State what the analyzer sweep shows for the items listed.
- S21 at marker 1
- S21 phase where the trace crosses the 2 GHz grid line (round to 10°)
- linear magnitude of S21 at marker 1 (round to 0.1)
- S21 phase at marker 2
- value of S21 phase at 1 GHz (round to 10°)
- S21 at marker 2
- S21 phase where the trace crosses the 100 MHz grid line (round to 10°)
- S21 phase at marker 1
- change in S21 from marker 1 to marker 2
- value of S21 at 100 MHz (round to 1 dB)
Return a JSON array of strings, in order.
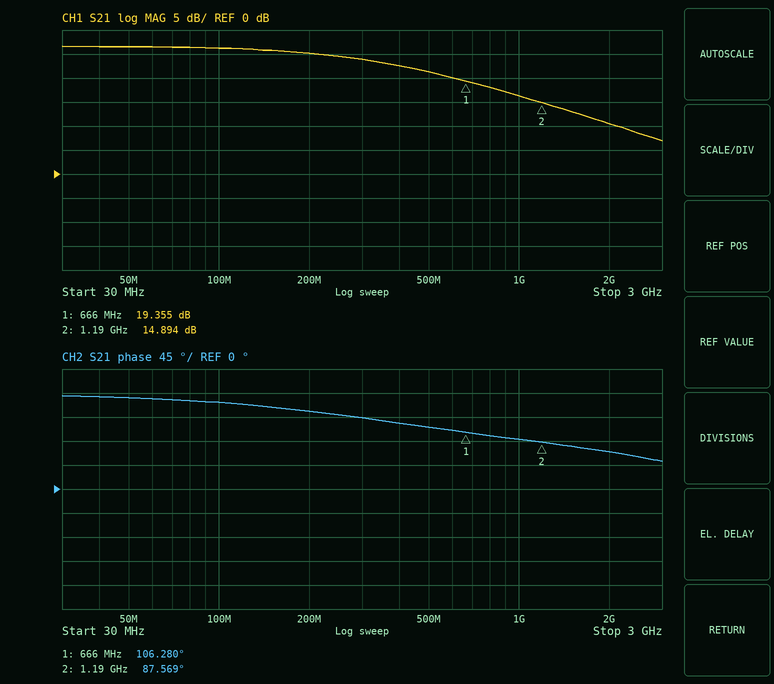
["19.355 dB", "70°", "9.3", "87.569°", "90°", "14.894 dB", "160°", "106.280°", "-4.461 dB", "26 dB"]
